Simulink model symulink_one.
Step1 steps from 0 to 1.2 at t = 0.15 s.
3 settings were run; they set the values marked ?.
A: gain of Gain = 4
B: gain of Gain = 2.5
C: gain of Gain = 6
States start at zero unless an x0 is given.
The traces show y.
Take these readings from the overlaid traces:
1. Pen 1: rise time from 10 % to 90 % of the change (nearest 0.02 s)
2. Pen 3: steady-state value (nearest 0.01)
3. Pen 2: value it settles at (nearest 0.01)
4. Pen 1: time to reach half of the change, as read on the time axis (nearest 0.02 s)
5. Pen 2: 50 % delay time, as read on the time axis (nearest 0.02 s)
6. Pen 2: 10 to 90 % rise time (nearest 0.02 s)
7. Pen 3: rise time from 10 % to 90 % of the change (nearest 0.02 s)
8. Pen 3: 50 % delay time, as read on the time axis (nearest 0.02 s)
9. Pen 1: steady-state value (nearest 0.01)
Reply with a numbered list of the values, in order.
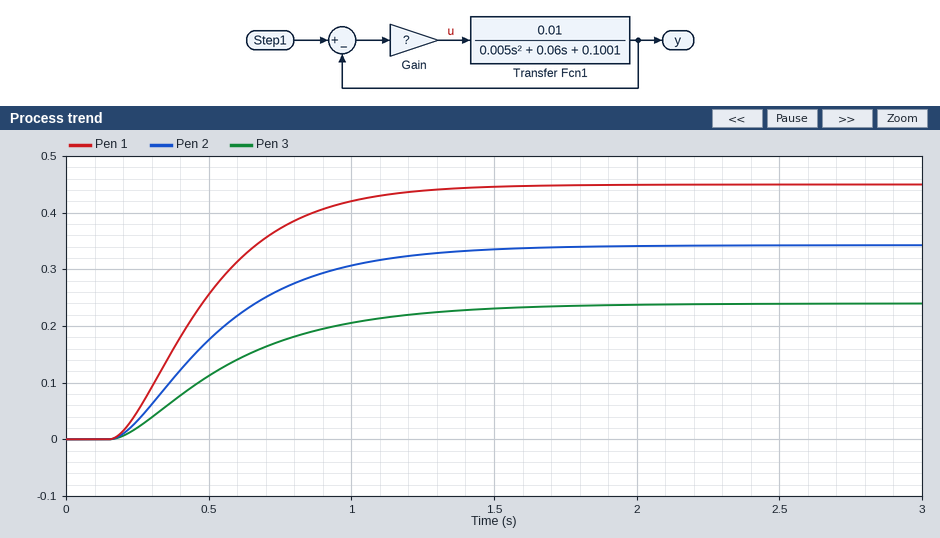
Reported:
1. 0.64 s
2. 0.24
3. 0.34
4. 0.46 s
5. 0.50 s
6. 0.76 s
7. 0.88 s
8. 0.52 s
9. 0.45
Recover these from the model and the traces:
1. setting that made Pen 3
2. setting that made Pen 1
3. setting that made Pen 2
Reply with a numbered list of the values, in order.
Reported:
1. B
2. C
3. A
